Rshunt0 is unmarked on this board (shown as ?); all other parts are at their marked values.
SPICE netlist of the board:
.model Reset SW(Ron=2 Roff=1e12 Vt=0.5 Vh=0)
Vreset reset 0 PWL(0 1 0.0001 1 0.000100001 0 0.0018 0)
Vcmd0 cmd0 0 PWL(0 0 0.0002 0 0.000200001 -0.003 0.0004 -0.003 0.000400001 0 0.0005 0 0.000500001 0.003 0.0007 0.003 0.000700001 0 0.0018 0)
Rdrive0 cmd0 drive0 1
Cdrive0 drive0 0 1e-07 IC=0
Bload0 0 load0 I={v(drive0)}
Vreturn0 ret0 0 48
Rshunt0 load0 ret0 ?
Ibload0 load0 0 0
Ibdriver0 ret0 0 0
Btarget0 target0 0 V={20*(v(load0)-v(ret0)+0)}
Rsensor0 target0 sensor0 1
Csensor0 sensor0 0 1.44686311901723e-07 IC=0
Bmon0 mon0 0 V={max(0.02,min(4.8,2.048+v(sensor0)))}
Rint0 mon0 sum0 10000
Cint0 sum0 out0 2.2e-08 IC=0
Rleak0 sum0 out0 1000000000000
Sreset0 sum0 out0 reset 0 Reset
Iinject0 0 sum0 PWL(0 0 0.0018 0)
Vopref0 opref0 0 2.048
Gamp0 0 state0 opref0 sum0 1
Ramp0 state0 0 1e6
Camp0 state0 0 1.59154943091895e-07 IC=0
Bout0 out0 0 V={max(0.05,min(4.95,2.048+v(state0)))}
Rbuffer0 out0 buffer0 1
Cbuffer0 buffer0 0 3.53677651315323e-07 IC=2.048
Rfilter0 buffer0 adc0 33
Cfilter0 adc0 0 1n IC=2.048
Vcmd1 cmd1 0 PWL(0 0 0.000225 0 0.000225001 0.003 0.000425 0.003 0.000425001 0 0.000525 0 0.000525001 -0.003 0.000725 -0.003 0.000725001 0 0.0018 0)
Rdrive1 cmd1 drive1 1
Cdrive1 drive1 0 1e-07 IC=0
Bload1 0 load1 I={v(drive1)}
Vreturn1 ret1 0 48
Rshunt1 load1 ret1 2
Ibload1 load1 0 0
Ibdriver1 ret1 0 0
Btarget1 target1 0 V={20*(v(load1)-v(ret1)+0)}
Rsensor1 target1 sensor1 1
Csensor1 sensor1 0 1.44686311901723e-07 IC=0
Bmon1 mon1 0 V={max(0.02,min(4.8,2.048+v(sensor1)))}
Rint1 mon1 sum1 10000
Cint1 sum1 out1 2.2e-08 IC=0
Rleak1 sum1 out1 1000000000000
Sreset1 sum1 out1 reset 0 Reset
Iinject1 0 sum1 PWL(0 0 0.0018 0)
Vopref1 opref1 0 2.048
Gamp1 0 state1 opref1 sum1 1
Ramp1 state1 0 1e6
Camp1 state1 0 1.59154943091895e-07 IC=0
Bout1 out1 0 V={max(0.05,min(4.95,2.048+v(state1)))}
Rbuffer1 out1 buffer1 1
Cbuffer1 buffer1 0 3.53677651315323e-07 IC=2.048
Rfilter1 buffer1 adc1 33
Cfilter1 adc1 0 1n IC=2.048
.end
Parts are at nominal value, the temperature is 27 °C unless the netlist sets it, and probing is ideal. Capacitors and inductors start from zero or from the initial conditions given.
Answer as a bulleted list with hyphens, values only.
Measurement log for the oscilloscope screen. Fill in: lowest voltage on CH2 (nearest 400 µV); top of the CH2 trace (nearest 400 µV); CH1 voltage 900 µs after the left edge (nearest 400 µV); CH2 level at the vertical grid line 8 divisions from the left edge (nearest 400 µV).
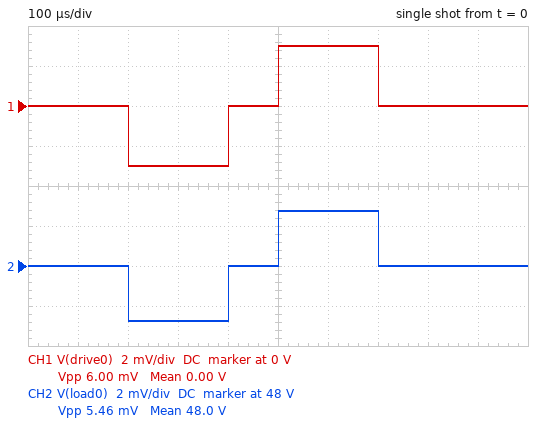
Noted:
- 47.9972 V
- 48.0028 V
- 0 V
- 48.0000 V
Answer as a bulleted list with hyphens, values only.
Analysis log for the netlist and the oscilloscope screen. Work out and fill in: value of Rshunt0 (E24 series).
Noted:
- 0.91 Ω
